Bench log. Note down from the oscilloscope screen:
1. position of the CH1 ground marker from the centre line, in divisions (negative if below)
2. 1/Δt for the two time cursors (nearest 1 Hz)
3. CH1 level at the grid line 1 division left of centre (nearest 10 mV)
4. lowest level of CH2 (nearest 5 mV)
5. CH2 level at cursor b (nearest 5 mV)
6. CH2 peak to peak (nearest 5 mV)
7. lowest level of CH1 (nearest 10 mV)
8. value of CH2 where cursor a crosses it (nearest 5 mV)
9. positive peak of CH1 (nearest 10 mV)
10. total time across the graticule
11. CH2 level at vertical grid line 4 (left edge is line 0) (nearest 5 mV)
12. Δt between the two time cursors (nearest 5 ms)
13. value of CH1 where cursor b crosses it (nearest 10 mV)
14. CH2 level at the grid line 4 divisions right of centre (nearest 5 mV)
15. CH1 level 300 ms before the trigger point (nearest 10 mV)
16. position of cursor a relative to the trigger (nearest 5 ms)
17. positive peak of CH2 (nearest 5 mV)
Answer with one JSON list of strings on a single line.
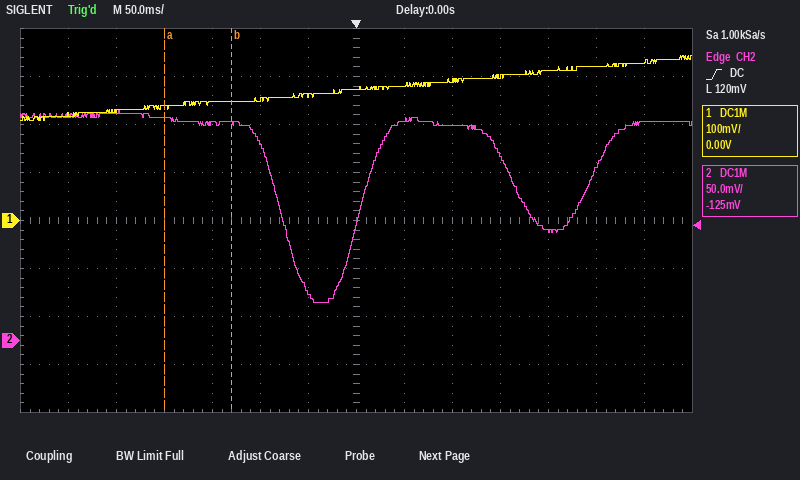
["0.0 div", "14 Hz", "260 mV", "40 mV", "225 mV", "200 mV", "210 mV", "230 mV", "340 mV", "700 ms", "225 mV", "70 ms", "250 mV", "115 mV", "220 mV", "-200 ms", "240 mV"]
